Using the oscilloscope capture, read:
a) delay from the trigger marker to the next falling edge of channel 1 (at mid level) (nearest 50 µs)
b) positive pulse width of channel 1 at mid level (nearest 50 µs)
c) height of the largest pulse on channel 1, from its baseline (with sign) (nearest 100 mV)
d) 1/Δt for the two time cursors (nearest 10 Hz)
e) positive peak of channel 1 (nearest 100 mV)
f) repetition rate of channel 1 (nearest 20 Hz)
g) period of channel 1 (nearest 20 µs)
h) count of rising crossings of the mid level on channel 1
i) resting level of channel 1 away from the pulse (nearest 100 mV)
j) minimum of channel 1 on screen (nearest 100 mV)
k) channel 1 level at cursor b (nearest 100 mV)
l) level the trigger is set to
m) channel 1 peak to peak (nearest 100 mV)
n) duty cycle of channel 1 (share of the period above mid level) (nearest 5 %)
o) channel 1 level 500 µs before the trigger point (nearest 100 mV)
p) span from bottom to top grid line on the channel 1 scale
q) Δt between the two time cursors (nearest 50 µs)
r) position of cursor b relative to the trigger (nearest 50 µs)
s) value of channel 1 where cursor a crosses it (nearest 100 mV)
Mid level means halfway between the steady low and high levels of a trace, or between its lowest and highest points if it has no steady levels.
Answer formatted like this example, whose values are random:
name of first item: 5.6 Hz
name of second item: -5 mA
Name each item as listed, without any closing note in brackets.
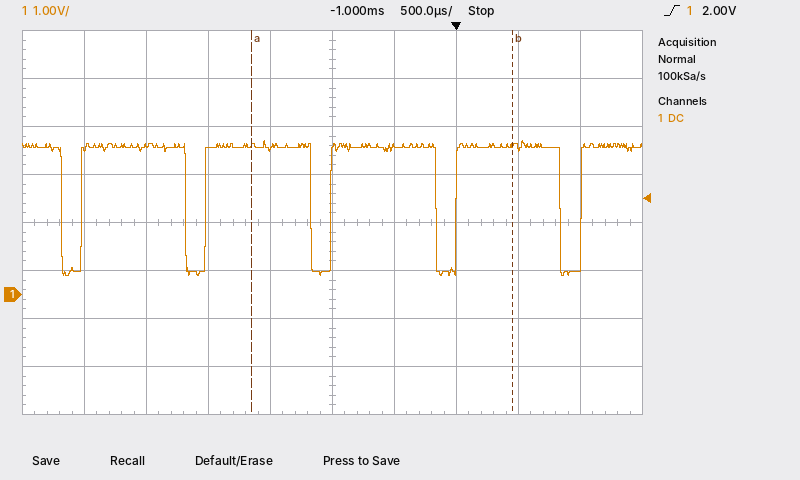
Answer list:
delay from the trigger marker to the next falling edge of channel 1 (at mid level): 850 µs
positive pulse width of channel 1 at mid level: 850 µs
height of the largest pulse on channel 1, from its baseline (with sign): -2.7 V
1/Δt for the two time cursors: 480 Hz
positive peak of channel 1: 3.2 V
repetition rate of channel 1: 1.00 kHz
period of channel 1: 1.00 ms
count of rising crossings of the mid level on channel 1: 5
resting level of channel 1 away from the pulse: 3.1 V
minimum of channel 1 on screen: 400 mV
channel 1 level at cursor b: 3.1 V
level the trigger is set to: 2.00 V
channel 1 peak to peak: 2.8 V
duty cycle of channel 1 (share of the period above mid level): 85 %
channel 1 level 500 µs before the trigger point: 3.1 V
span from bottom to top grid line on the channel 1 scale: 8 V
Δt between the two time cursors: 2.10 ms
position of cursor b relative to the trigger: +450 µs
value of channel 1 where cursor a crosses it: 3.1 V
